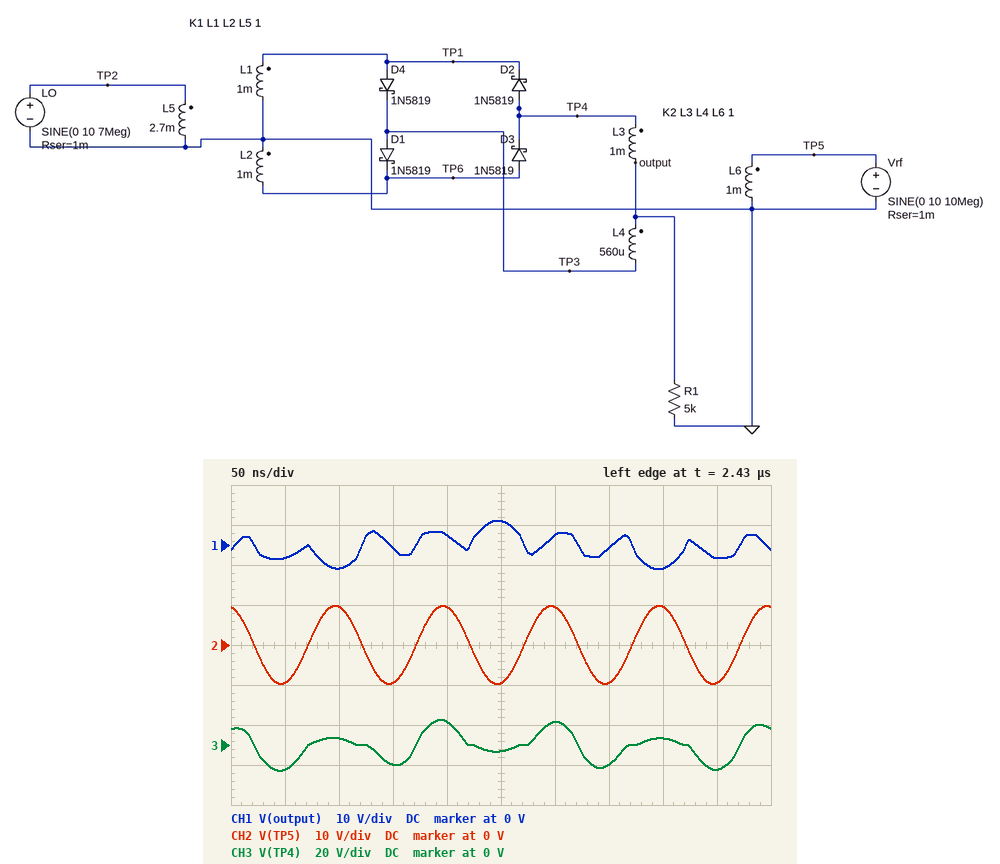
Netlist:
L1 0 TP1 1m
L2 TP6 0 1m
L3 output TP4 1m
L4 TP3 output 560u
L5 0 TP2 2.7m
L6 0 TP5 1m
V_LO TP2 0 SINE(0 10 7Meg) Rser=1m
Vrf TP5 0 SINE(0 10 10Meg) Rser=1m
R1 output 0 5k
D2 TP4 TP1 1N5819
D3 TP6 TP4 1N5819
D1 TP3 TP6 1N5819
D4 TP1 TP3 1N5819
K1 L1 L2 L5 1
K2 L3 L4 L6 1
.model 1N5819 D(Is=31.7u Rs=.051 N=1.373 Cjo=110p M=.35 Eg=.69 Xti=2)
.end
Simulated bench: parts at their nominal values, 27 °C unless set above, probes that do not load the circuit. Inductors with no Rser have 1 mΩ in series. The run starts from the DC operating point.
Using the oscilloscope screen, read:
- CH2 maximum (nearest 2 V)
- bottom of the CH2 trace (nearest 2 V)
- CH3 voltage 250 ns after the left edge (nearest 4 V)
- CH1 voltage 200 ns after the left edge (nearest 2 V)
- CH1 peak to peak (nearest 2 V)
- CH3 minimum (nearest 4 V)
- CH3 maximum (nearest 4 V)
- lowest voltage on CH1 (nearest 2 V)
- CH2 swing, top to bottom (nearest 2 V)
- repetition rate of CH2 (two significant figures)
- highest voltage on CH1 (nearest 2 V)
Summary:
10 V
-10 V
-4 V
2 V
12 V
-12 V
12 V
-6 V
20 V
10 MHz
6 V
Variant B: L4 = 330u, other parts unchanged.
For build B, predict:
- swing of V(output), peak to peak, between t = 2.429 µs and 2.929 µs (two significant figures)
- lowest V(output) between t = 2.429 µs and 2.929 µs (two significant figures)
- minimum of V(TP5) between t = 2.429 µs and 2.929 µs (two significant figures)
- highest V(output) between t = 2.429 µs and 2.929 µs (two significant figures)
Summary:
13 V
-6.7 V
-9.8 V
6.7 V
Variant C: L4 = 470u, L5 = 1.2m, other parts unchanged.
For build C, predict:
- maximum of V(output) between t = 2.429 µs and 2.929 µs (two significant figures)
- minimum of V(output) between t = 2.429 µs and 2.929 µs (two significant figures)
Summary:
7.2 V
-7.2 V
